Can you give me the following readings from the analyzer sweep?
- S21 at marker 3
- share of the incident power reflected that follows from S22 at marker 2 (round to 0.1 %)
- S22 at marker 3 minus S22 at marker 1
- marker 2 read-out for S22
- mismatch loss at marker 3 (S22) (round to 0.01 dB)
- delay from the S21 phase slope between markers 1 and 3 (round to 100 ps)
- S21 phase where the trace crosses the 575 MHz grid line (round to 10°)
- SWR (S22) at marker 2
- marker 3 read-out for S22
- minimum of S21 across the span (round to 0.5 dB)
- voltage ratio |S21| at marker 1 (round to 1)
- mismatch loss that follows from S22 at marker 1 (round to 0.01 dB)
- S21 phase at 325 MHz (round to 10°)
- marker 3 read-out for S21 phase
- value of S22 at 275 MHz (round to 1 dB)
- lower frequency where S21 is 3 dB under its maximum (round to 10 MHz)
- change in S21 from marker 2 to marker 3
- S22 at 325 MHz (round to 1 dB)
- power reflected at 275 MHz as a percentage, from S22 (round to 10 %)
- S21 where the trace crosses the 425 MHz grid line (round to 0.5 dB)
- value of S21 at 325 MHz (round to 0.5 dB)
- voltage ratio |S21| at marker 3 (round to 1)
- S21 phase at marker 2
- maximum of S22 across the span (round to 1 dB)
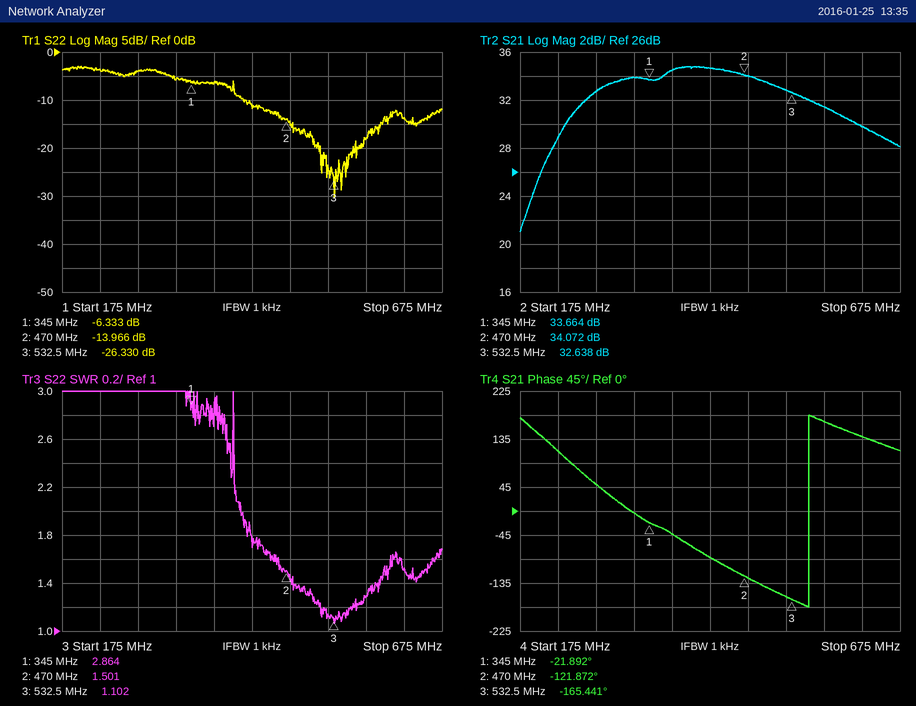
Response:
32.638 dB
4.0 %
-19.997 dB
-13.966 dB
0.01 dB
2.1 ns
170°
1.501
-26.330 dB
21.0 dB
48
1.15 dB
0°
-165.441°
-4 dB
260 MHz
-1.434 dB
-6 dB
40 %
34.5 dB
34.0 dB
43
-121.872°
-3 dB
